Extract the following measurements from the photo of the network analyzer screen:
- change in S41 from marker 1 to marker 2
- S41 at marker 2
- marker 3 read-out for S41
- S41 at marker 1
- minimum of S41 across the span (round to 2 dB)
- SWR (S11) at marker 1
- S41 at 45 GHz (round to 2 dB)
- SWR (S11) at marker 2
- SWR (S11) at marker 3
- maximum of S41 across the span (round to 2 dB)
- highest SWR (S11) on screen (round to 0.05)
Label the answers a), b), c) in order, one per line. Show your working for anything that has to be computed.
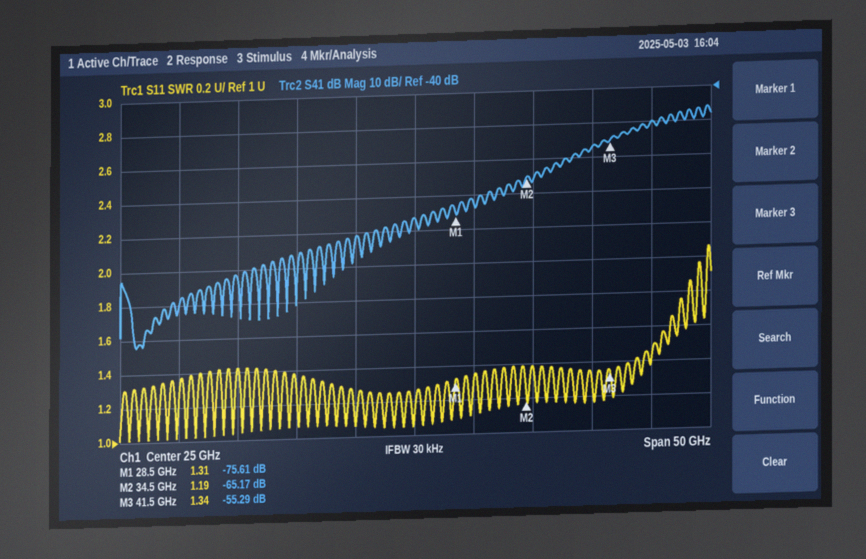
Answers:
a) -65.17 − (-75.61) = 10.44 dB
b) -65.17 dB
c) -55.29 dB
d) -75.61 dB
e) -112 dB
f) 1.31
g) -50 dB
h) 1.19
i) 1.34
j) -46 dB
k) 2.05
